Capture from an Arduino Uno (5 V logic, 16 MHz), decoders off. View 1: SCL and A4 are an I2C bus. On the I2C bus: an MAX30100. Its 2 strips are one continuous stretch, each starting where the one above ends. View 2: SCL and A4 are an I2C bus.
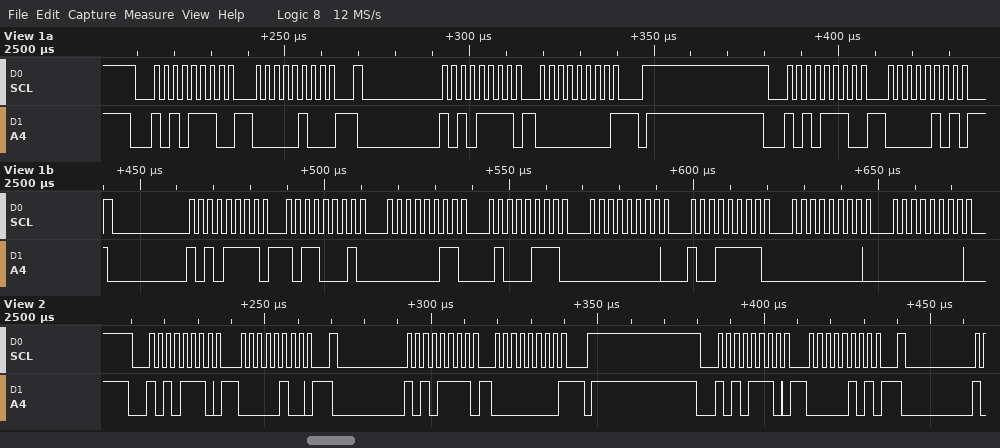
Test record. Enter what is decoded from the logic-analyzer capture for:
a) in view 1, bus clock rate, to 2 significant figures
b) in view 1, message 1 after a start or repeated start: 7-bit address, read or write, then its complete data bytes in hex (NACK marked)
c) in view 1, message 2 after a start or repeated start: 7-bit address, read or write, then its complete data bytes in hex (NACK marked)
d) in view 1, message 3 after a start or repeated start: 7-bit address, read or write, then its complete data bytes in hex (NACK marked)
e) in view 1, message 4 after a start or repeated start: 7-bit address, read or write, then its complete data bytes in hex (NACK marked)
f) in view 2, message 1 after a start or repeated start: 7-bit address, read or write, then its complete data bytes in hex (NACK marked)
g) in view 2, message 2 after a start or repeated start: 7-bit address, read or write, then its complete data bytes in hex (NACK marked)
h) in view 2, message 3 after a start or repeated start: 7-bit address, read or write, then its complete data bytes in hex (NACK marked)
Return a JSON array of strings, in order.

["400 kHz", "0x57 write: 04", "0x57 read: 00 NACK", "0x57 write: 05", "0x57 read: B1 03 47 00 9F 00 00", "0x57 write: 04", "0x57 read: 00 NACK", "0x57 write: 05"]
